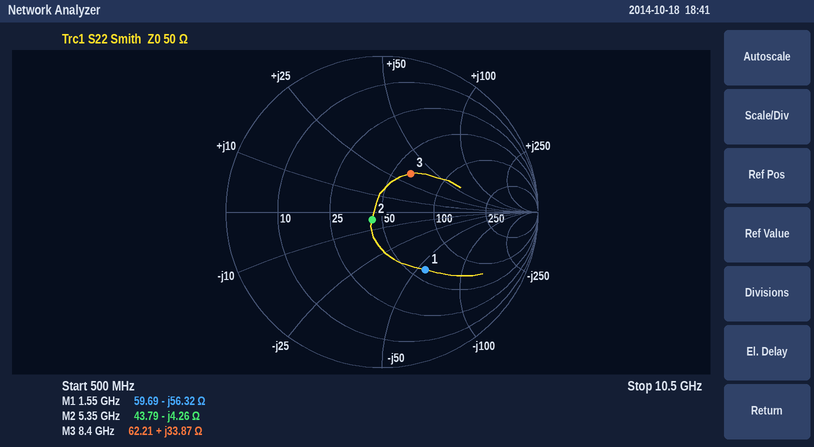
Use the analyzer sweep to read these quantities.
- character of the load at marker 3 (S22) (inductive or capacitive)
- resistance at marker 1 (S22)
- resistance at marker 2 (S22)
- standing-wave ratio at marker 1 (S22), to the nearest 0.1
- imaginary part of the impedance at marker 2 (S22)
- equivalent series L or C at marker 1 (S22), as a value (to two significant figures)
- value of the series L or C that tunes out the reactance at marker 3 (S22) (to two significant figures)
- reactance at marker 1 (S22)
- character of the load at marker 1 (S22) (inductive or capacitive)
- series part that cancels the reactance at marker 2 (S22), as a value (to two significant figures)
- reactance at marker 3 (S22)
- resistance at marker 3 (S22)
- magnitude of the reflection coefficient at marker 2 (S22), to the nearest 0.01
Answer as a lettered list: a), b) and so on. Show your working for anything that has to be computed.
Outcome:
a) inductive
b) 59.69 Ω
c) 43.79 Ω
d) 2.7
e) -4.26 Ω
f) C = 1/(2π × 1.55 GHz × 56.32 Ω) ≈ 1.8 pF
g) C = 1/(2π × 8.4 GHz × 33.87 Ω) ≈ 559 fF, so 560 fF to two significant figures
h) -56.32 Ω
i) capacitive
j) L = 4.26 Ω/(2π × 5.35 GHz) ≈ 127 pH, so 130 pH to two significant figures
k) +33.87 Ω
l) 62.21 Ω
m) 0.08
